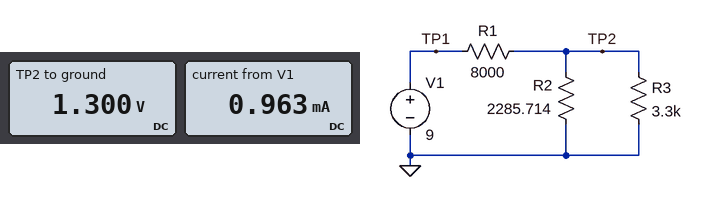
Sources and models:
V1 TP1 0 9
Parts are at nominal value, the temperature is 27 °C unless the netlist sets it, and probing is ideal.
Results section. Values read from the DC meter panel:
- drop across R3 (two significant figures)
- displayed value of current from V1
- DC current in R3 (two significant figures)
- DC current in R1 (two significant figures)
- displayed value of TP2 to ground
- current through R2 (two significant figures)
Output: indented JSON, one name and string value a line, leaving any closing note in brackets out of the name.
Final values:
{
  "drop across R3": "1.3 V",
  "displayed value of current from V1": "0.963 mA",
  "DC current in R3": "390 µA",
  "DC current in R1": "960 µA",
  "displayed value of TP2 to ground": "1.300 V",
  "current through R2": "570 µA"
}
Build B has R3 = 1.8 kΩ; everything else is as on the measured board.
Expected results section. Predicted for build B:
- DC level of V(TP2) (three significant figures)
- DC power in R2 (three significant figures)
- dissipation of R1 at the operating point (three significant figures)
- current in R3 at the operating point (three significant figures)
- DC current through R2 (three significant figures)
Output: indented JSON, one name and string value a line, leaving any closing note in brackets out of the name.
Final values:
{
  "DC level of V(TP2)": "1.01 V",
  "DC power in R2": "443 µW",
  "dissipation of R1 at the operating point": "7.99 mW",
  "current in R3 at the operating point": "559 µA",
  "DC current through R2": "440 µA"
}
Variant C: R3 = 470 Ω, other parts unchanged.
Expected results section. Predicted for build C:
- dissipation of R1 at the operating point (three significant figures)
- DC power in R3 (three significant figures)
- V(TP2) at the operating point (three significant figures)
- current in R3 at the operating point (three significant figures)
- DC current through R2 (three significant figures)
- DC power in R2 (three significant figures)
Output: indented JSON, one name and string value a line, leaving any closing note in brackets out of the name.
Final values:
{
  "dissipation of R1 at the operating point": "9.21 mW",
  "DC power in R3": "372 µW",
  "V(TP2) at the operating point": "418 mV",
  "current in R3 at the operating point": "890 µA",
  "DC current through R2": "183 µA",
  "DC power in R2": "76.5 µW"
}
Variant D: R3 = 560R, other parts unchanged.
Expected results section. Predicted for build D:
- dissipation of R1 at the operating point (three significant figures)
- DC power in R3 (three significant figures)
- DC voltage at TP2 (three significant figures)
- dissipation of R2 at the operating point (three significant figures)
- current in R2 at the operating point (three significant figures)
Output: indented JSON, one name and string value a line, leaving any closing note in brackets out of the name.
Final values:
{
  "dissipation of R1 at the operating point": "9.08 mW",
  "DC power in R3": "410 µW",
  "DC voltage at TP2": "479 mV",
  "dissipation of R2 at the operating point": "100 µW",
  "current in R2 at the operating point": "210 µA"
}
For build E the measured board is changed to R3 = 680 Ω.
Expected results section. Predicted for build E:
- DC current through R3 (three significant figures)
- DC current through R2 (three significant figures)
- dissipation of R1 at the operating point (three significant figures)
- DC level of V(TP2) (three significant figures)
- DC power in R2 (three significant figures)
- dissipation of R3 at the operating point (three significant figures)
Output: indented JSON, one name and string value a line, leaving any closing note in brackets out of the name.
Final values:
{
  "DC current through R3": "814 µA",
  "DC current through R2": "242 µA",
  "dissipation of R1 at the operating point": "8.92 mW",
  "DC level of V(TP2)": "553 mV",
  "DC power in R2": "134 µW",
  "dissipation of R3 at the operating point": "450 µW"
}
